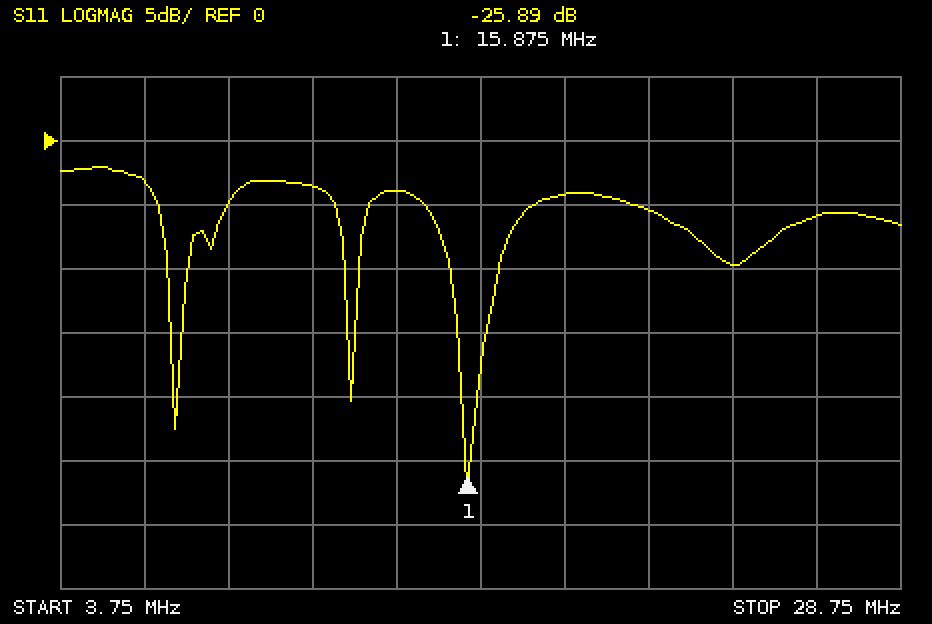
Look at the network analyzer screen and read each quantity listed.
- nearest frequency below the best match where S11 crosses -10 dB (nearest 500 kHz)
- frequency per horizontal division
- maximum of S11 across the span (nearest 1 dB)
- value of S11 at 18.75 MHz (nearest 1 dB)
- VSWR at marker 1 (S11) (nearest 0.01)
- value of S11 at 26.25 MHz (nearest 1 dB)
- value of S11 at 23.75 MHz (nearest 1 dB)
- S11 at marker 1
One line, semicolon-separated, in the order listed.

15.5 MHz; 2.5 MHz; -2 dB; -4 dB; 1.11; -6 dB; -10 dB; -25.89 dB
